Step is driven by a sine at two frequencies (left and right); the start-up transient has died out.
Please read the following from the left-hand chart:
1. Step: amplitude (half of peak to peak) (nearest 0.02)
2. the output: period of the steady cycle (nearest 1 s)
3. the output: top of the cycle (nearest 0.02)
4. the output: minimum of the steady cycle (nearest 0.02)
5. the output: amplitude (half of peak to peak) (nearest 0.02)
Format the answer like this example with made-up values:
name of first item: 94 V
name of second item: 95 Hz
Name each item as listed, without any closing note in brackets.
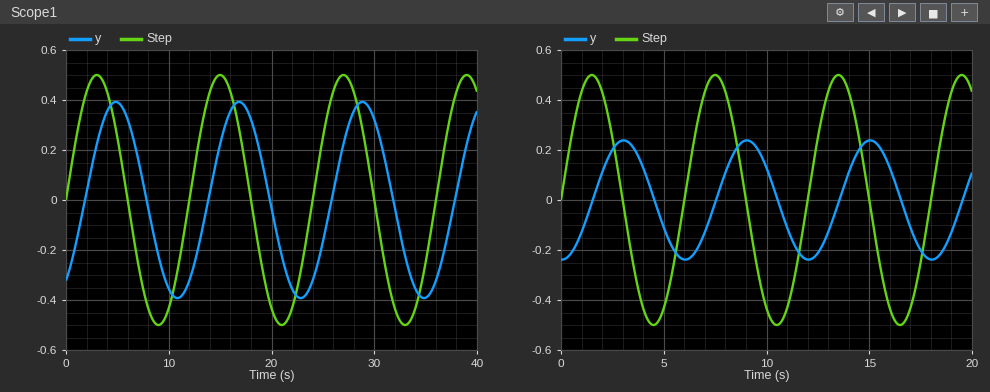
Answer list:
Step: amplitude (half of peak to peak): 0.50
the output: period of the steady cycle: 12 s
the output: top of the cycle: 0.40
the output: minimum of the steady cycle: -0.40
the output: amplitude (half of peak to peak): 0.40
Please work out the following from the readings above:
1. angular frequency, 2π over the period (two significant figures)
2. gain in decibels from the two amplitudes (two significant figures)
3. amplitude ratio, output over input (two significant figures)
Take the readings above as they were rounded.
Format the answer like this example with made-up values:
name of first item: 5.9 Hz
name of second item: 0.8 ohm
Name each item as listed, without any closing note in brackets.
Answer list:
angular frequency, 2π over the period: 0.52 rad/s
gain in decibels from the two amplitudes: -1.9 dB
amplitude ratio, output over input: 0.80
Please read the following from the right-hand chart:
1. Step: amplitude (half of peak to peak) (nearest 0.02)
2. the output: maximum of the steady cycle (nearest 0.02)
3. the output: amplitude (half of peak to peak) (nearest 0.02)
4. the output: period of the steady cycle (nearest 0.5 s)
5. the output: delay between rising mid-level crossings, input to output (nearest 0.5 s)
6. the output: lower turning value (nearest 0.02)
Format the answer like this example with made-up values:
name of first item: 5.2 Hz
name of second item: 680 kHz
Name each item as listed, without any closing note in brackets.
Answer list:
Step: amplitude (half of peak to peak): 0.50
the output: maximum of the steady cycle: 0.24
the output: amplitude (half of peak to peak): 0.24
the output: period of the steady cycle: 6.0 s
the output: delay between rising mid-level crossings, input to output: 1.5 s
the output: lower turning value: -0.24
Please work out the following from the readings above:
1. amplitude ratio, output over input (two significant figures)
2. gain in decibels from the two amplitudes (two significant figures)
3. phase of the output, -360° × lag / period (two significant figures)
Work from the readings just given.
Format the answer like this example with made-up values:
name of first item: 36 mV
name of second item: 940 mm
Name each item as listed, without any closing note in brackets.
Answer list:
amplitude ratio, output over input: 0.48
gain in decibels from the two amplitudes: -6.4 dB
phase of the output, -360° × lag / period: -90°
